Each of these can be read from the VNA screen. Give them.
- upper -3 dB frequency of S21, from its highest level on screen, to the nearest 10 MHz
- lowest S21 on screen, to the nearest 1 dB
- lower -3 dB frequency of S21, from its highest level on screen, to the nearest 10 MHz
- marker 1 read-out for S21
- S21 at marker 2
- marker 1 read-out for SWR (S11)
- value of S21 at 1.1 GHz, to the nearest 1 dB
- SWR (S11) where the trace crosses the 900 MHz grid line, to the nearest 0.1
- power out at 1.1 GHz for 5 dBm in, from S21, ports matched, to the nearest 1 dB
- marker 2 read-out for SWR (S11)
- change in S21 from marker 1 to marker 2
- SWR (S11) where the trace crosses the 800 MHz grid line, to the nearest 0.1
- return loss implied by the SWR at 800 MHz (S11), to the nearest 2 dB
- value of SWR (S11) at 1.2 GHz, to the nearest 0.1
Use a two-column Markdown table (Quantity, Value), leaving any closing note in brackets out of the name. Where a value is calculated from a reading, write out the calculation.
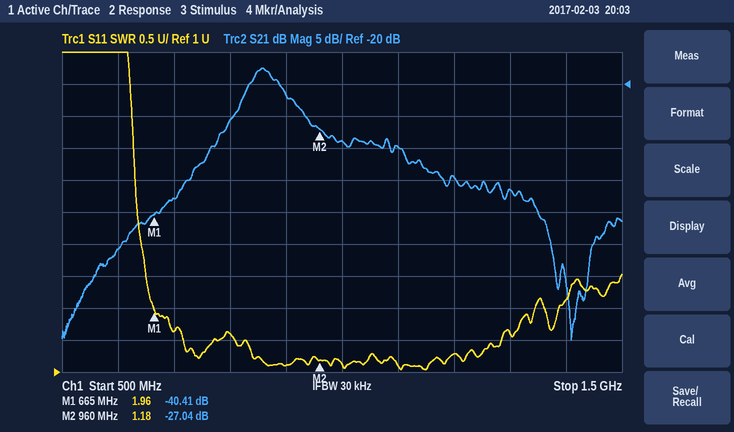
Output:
| Quantity | Value |
|---|---|
| upper -3 dB frequency of S21, from its highest level on screen, to the nearest 10 MHz | 890 MHz |
| lowest S21 on screen, to the nearest 1 dB | -60 dB |
| lower -3 dB frequency of S21, from its highest level on screen, to the nearest 10 MHz | 830 MHz |
| marker 1 read-out for S21 | -40.41 dB |
| S21 at marker 2 | -27.04 dB |
| marker 1 read-out for SWR | 1.96 |
| value of S21 at 1.1 GHz, to the nearest 1 dB | -30 dB |
| SWR (S11) where the trace crosses the 900 MHz grid line, to the nearest 0.1 | 1.1 |
| power out at 1.1 GHz for 5 dBm in, from S21, ports matched, to the nearest 1 dB | 5 dBm + (-30 dB) = -25 dBm |
| marker 2 read-out for SWR | 1.18 |
| change in S21 from marker 1 to marker 2 | -27.04 − (-40.41) = 13.37 dB |
| SWR (S11) where the trace crosses the 800 MHz grid line, to the nearest 0.1 | 1.6 |
| return loss implied by the SWR at 800 MHz (S11), to the nearest 2 dB | −20 log10((1.6 − 1)/(1.6 + 1)) ≈ 12.7 dB, so 12 dB to the nearest 2 dB |
| value of SWR (S11) at 1.2 GHz, to the nearest 0.1 | 1.3 |
